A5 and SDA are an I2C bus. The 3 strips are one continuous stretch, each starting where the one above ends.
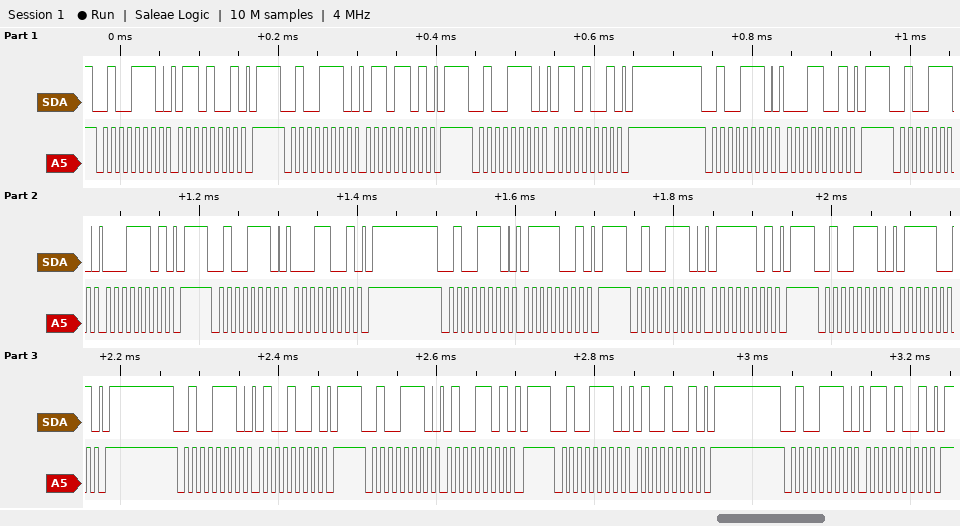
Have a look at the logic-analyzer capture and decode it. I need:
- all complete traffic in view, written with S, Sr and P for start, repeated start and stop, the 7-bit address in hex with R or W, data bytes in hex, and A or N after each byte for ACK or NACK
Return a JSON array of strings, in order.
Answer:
["S 27W A 69 A P S 27W A 6D A P S 27W A 69 A P S 27W A 19 A P S 27W A 1D A P S 27W A 19 A P S 27W A 79 A P S 27W A 7D A P S 27W A 79 A P S 27W A 49 A P S 27W A 4D A P S 27W A 49 A P S 27W A 69 A P"]
